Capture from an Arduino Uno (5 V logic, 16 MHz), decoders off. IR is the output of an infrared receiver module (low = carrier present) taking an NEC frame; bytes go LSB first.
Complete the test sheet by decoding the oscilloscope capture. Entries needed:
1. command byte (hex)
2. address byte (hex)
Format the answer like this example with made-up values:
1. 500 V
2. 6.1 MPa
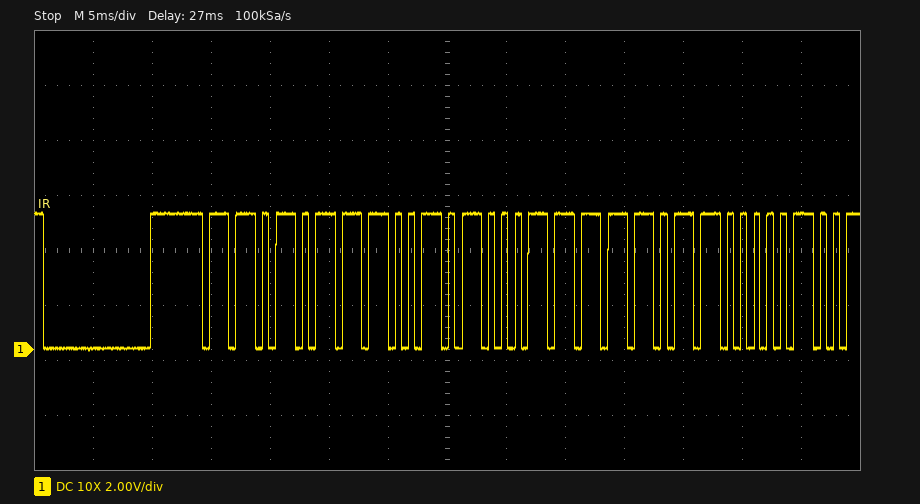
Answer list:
1. 0xDF
2. 0xEB
